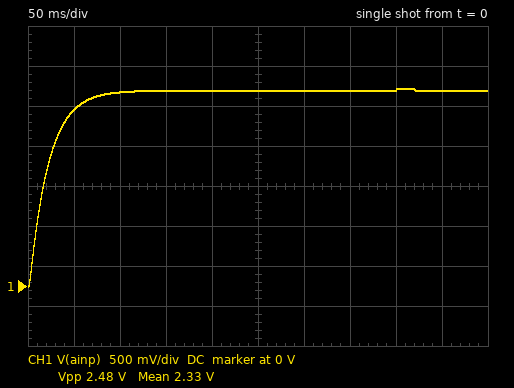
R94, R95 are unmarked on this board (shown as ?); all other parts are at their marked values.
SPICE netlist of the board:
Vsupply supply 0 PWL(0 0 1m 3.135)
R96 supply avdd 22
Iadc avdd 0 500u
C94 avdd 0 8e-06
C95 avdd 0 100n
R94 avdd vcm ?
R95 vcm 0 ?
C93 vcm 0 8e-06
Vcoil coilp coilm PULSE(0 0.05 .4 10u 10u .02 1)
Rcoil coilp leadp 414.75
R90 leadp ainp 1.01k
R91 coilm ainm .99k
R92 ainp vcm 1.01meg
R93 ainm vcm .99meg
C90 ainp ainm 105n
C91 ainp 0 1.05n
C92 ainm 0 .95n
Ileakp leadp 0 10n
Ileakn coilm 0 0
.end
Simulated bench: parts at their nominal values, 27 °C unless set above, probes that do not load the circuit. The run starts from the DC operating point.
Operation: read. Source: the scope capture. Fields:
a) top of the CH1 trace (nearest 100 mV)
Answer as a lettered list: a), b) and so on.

a) 2.5 V
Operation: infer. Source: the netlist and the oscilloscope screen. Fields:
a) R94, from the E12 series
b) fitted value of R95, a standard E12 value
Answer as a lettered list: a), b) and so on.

a) 3.3 kΩ
b) 12 kΩ
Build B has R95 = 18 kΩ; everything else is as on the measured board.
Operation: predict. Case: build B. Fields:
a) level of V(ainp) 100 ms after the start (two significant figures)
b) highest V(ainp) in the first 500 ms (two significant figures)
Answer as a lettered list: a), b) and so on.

a) 2.6 V
b) 2.7 V
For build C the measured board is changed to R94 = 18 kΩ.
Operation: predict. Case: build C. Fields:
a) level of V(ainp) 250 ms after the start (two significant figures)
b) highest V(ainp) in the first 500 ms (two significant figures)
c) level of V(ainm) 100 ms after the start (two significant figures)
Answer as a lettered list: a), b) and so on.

a) 1.2 V
b) 1.3 V
c) 1.0 V
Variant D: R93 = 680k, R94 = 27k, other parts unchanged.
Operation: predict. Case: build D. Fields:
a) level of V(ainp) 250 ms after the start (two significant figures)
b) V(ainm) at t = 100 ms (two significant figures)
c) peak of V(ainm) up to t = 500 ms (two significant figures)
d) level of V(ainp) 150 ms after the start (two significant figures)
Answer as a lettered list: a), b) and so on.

a) 930 mV
b) 740 mV
c) 960 mV
d) 850 mV
